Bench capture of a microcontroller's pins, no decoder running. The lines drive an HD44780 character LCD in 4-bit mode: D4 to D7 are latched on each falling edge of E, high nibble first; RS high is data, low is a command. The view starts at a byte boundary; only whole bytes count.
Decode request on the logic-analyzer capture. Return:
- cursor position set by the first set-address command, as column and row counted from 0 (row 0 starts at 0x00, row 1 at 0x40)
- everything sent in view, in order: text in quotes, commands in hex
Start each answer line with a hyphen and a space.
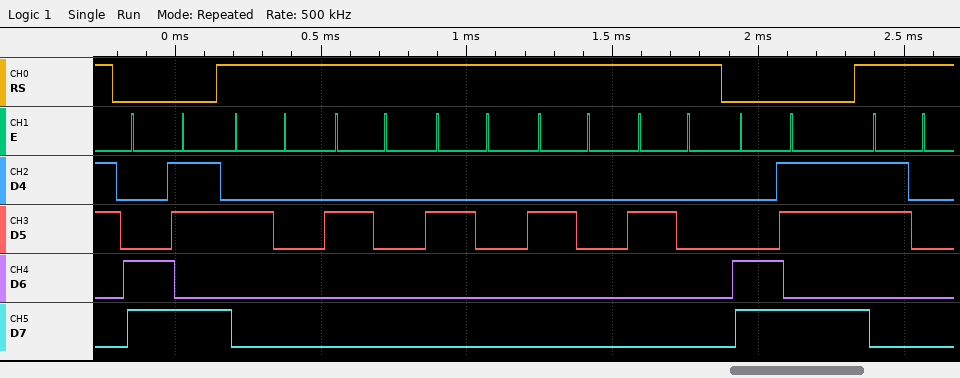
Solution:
- column 11, row 1
- 0xCB "     " 0xCB "0"
